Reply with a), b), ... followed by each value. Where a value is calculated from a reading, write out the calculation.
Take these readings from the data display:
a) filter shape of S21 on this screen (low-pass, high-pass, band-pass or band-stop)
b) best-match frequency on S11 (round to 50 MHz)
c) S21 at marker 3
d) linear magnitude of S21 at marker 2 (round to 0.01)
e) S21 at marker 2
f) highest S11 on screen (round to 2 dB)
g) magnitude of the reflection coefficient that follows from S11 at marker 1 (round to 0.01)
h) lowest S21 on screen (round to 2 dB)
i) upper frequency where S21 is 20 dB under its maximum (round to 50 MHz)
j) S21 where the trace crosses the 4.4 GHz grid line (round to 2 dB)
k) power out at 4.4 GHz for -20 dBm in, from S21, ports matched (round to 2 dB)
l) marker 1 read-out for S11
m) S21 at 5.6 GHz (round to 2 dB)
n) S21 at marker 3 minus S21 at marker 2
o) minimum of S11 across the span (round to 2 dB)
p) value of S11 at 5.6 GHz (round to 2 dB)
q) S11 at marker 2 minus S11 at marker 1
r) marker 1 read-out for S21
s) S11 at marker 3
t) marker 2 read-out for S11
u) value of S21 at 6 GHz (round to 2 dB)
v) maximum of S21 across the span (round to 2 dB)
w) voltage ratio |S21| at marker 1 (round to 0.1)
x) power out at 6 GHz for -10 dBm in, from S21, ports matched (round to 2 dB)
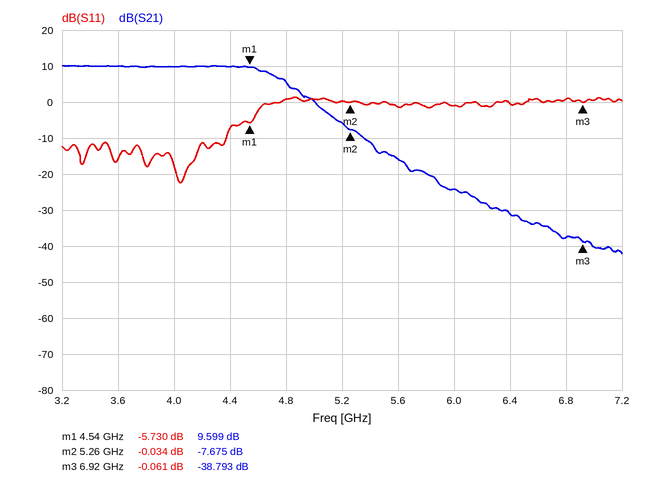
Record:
a) low-pass
b) 4.05 GHz
c) -38.793 dB
d) 10^(-7.675/20) ≈ 0.41
e) -7.675 dB
f) 2 dB
g) 10^(-5.73/20) ≈ 0.52
h) -42 dB
i) 5.35 GHz
j) 10 dB
k) -20 dBm + (10 dB) = -10 dBm
l) -5.730 dB
m) -16 dB
n) -38.793 − (-7.675) = -31.118 dB
o) -22 dB
p) -2 dB
q) -0.034 − (-5.73) = 5.696 dB
r) 9.599 dB
s) -0.061 dB
t) -0.034 dB
u) -24 dB
v) 10 dB
w) 10^(9.599/20) ≈ 3.0
x) -10 dBm + (-24 dB) = -34 dBm
